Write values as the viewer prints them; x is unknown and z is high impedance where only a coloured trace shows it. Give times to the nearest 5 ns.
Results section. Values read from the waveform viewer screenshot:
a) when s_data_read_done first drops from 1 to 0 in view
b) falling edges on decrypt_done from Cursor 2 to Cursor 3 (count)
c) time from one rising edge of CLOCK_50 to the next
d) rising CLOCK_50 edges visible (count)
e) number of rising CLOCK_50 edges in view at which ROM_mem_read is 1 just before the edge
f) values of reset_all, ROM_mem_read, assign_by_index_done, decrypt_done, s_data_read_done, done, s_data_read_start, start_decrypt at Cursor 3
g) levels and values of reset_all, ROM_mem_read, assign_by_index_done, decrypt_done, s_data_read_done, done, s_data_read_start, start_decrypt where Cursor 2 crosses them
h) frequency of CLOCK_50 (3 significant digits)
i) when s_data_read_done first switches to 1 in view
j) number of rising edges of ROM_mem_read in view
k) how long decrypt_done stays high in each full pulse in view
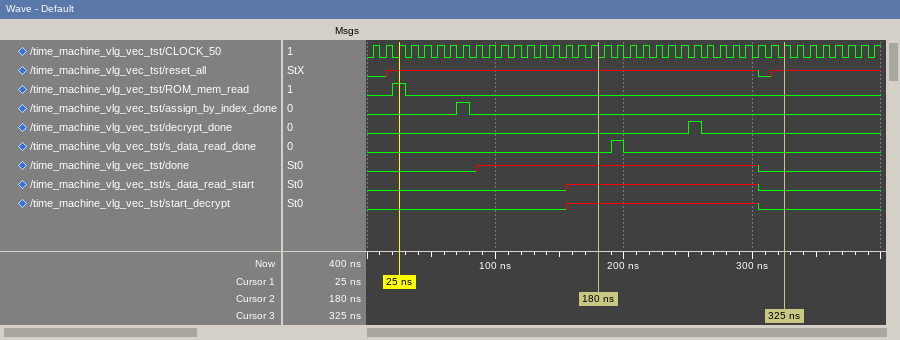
200 ns
1
10 ns
40
1
reset_all=x, ROM_mem_read=0, assign_by_index_done=0, decrypt_done=0, s_data_read_done=0, done=0, s_data_read_start=0, start_decrypt=0
reset_all=x, ROM_mem_read=0, assign_by_index_done=0, decrypt_done=0, s_data_read_done=0, done=x, s_data_read_start=x, start_decrypt=x
100 MHz
190 ns
1
10 ns
